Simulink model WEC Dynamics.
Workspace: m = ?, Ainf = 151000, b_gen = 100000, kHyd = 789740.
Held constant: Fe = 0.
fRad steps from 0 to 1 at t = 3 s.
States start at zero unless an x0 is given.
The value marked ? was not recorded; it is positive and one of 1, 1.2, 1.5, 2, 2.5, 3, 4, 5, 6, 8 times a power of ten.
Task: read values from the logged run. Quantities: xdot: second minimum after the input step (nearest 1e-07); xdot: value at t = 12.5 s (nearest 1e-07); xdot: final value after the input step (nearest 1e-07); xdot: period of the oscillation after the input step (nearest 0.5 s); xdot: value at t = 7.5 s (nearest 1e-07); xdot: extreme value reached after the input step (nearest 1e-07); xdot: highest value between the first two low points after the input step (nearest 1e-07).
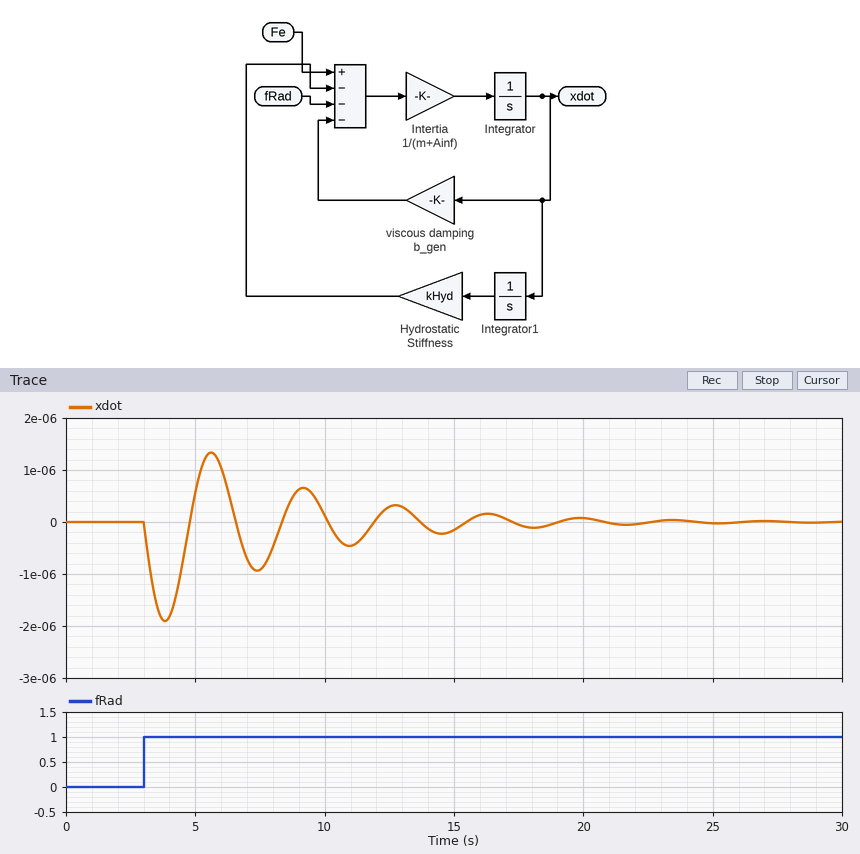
-0.0000009
0.0000003
0.0000000
3.5 s
-0.0000009
-0.0000019
0.0000013
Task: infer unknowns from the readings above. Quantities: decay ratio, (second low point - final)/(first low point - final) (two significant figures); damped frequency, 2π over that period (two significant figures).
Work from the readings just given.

0.47
1.8 rad/s
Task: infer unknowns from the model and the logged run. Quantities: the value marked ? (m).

100000
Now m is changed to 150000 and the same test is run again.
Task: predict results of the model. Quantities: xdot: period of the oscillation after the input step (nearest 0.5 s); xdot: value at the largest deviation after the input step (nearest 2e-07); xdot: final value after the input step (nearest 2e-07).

4.0 s
-0.0000018
0.0000000
